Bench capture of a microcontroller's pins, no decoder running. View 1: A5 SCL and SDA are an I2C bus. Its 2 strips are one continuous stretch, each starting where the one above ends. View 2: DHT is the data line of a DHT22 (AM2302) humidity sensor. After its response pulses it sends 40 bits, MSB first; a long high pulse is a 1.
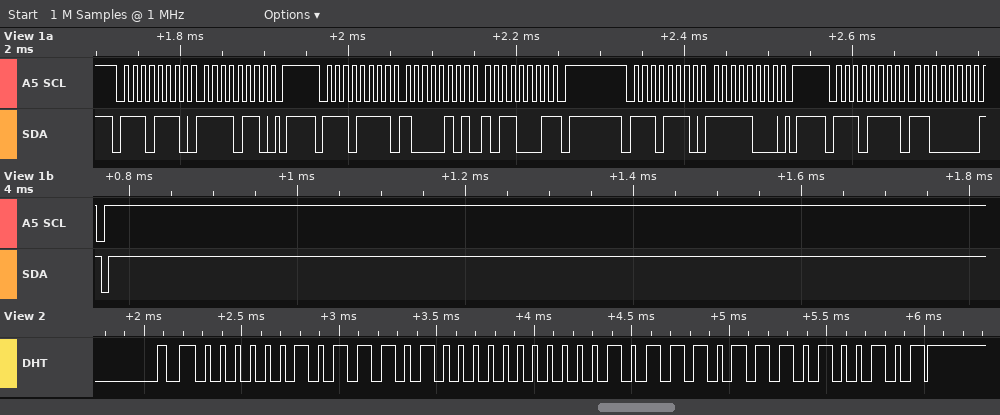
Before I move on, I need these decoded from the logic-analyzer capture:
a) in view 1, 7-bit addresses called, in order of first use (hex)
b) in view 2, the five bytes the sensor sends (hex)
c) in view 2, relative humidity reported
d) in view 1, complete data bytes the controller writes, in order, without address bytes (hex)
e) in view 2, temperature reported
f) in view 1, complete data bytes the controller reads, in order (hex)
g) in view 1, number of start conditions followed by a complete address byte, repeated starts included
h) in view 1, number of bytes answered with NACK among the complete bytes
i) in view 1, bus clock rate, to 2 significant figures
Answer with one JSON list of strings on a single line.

["0x77", "02 E8 00 BB A5", "74.4 %", "F6 F8", "18.7 °C", "85 B1 C0", "4", "2", "100 kHz"]
